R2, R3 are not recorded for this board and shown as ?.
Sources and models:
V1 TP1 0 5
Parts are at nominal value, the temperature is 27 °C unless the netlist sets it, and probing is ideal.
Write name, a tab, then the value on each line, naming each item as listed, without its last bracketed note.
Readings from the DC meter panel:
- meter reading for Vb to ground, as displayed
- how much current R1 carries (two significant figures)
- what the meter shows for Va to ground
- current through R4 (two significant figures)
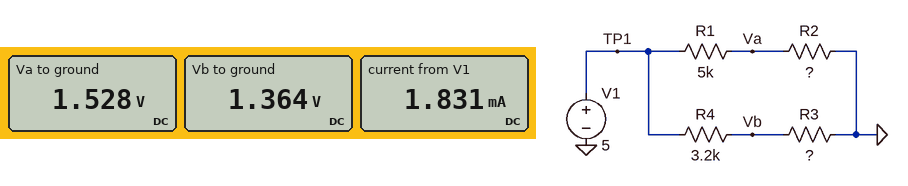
meter reading for Vb to ground, as displayed	1.364 V
how much current R1 carries	690 µA
what the meter shows for Va to ground	1.528 V
current through R4	1.1 mA
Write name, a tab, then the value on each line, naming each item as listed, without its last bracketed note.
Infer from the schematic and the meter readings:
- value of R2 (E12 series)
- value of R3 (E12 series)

value of R2	2.2 kΩ
value of R3	1.2 kΩ
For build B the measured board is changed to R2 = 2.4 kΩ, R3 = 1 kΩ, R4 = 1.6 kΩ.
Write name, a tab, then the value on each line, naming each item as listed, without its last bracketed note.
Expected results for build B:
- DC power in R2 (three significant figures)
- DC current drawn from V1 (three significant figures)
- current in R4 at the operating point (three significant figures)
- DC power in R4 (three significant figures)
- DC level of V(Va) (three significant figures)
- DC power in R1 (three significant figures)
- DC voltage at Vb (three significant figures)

DC power in R2	1.10 mW
DC current drawn from V1	2.60 mA
current in R4 at the operating point	1.92 mA
DC power in R4	5.92 mW
DC level of V(Va)	1.62 V
DC power in R1	2.28 mW
DC voltage at Vb	1.92 V
